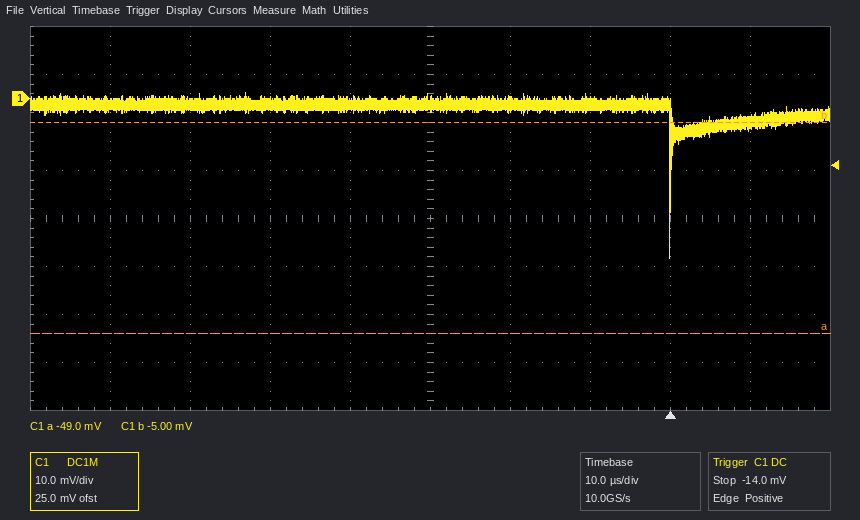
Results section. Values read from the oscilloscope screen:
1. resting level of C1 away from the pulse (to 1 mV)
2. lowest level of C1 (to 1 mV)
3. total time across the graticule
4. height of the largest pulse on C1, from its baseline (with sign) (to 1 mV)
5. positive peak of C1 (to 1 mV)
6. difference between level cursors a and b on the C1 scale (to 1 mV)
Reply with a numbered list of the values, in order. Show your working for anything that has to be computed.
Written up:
1. -1 mV
2. -33 mV
3. 100 µs
4. -33 mV − (-1 mV) = -32 mV
5. 1 mV
6. 44 mV
